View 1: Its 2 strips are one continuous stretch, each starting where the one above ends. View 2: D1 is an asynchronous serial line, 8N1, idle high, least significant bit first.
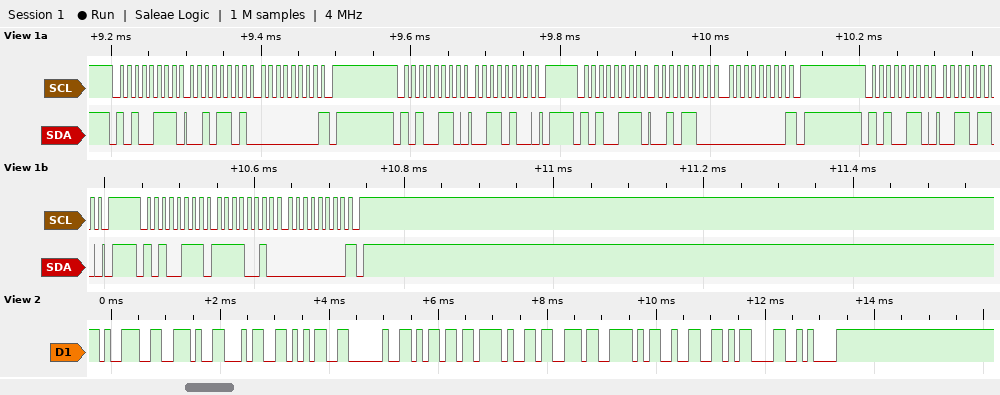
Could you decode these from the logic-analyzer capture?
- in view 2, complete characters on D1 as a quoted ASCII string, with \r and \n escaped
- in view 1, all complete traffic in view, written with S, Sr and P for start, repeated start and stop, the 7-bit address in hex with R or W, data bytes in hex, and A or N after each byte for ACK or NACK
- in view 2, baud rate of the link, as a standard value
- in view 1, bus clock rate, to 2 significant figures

"9.45 m/s^2\r\n"
S 53R A 2D A 00 N P S 53W A 34 A P S 53R A 2C A 00 N P S 53W A 36 A P S 53R A F2 A 00 N P
9600 baud
100 kHz
